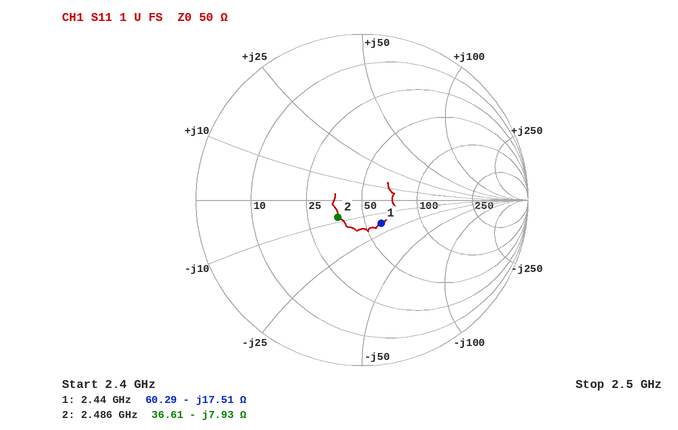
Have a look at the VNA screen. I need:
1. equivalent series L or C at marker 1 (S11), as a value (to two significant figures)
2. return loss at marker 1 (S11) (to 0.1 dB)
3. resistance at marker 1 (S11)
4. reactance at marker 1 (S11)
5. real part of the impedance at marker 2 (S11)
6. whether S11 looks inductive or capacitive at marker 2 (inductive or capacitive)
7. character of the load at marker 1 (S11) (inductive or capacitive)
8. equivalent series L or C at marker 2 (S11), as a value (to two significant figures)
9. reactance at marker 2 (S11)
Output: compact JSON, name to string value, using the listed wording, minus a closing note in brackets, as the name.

{"equivalent series L or C at marker 1 (S11), as a value": "3.7 pF", "return loss at marker 1 (S11)": "14.8 dB", "resistance at marker 1": "60.29 Ω", "reactance at marker 1": "-17.51 Ω", "real part of the impedance at marker 2": "36.61 Ω", "whether S11 looks inductive or capacitive at marker 2": "capacitive", "character of the load at marker 1 (S11)": "capacitive", "equivalent series L or C at marker 2 (S11), as a value": "8.1 pF", "reactance at marker 2": "-7.93 Ω"}
